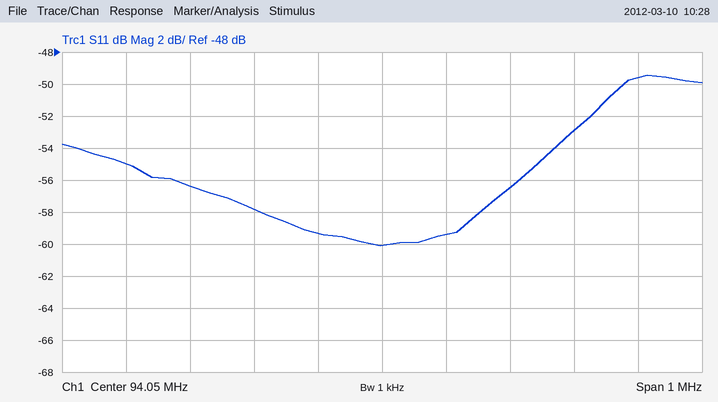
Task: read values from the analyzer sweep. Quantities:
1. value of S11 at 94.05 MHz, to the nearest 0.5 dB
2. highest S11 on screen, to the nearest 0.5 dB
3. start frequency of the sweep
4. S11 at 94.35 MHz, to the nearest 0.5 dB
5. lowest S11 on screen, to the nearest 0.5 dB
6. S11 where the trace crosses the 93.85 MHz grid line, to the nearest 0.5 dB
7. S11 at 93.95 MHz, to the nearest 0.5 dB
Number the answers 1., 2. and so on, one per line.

1. -60.0 dB
2. -49.5 dB
3. 93.55 MHz
4. -53.0 dB
5. -60.0 dB
6. -58.0 dB
7. -59.5 dB
